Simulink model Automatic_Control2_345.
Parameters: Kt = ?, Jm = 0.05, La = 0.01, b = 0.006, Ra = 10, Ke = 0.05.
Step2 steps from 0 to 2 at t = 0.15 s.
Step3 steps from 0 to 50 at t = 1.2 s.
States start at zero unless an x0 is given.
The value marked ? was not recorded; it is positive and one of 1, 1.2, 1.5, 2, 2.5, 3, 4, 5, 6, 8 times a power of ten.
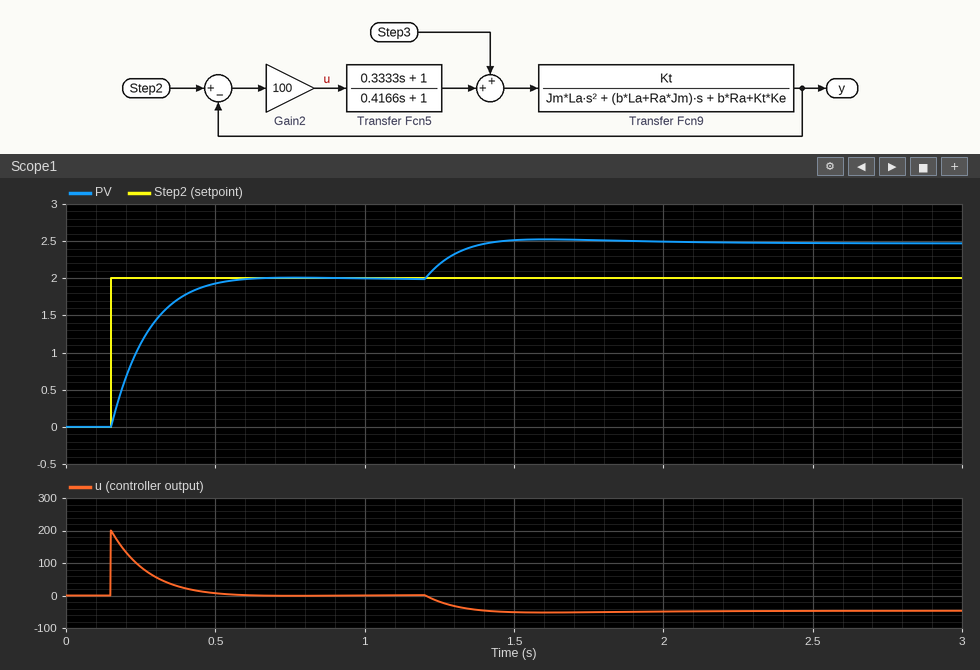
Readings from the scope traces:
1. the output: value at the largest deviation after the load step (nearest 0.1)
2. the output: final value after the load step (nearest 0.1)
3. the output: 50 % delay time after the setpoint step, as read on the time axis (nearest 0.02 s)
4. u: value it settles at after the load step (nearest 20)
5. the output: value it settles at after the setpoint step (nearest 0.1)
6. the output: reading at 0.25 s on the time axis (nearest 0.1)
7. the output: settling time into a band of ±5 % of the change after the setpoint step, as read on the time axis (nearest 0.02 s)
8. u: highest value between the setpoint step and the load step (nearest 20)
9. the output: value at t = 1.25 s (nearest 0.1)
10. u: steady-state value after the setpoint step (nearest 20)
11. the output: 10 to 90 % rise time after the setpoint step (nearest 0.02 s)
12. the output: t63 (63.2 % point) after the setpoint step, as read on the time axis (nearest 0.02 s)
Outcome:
2.5
2.5
0.24 s
-40
2.0
1.1
0.46 s
200
2.2
0
0.24 s
0.26 s
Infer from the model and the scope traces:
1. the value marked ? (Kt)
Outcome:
0.05
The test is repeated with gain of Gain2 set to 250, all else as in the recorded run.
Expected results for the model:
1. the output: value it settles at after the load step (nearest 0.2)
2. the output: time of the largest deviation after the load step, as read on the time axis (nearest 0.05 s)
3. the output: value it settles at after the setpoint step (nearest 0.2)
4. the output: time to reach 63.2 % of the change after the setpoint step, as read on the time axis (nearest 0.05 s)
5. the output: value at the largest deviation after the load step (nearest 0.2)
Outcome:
2.2
1.40 s
2.0
0.20 s
2.2
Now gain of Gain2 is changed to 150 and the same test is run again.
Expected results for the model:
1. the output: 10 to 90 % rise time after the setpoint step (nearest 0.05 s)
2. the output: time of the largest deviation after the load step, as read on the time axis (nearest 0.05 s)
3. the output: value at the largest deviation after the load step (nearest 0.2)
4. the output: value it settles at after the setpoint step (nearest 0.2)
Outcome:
0.15 s
1.50 s
2.4
2.0
